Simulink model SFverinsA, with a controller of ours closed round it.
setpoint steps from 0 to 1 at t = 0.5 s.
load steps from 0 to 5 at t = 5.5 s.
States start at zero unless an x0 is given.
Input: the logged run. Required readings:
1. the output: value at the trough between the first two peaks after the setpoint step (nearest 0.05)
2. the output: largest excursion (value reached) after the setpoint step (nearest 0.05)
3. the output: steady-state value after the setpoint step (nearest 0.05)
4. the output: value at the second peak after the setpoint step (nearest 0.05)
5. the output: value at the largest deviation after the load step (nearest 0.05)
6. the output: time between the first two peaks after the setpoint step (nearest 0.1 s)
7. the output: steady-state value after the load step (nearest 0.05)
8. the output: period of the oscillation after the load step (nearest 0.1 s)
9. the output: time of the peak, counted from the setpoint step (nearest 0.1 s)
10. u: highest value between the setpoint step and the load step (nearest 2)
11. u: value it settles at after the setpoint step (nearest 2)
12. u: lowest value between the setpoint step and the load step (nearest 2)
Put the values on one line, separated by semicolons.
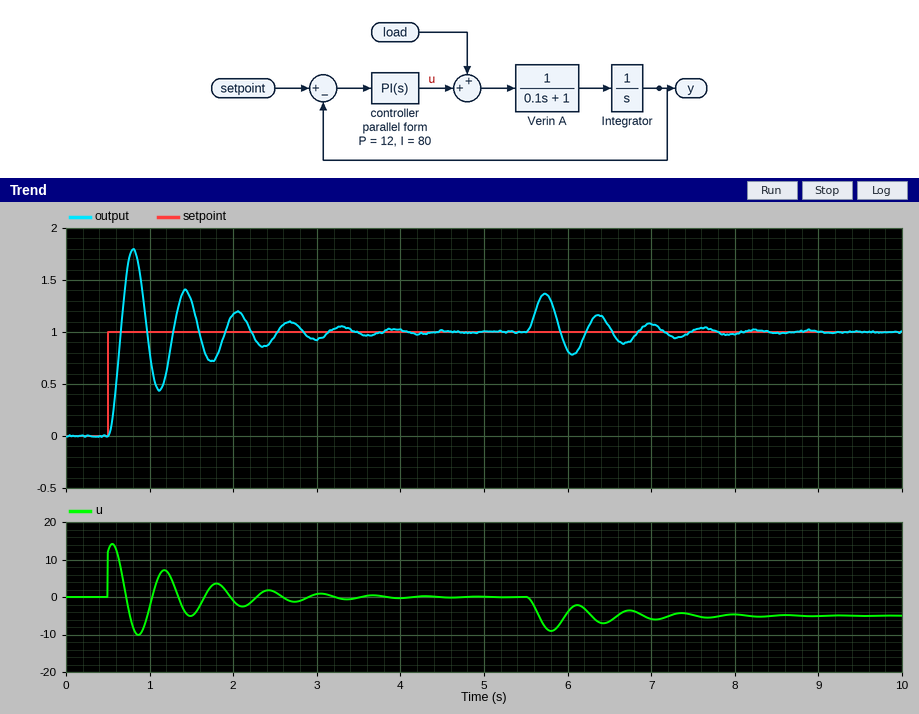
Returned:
0.45; 1.80; 1.00; 1.40; 1.35; 0.6 s; 1.00; 0.6 s; 0.3 s; 14; 0; -10
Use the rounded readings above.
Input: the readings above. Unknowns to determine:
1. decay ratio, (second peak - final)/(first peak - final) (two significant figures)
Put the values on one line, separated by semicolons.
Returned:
0.50
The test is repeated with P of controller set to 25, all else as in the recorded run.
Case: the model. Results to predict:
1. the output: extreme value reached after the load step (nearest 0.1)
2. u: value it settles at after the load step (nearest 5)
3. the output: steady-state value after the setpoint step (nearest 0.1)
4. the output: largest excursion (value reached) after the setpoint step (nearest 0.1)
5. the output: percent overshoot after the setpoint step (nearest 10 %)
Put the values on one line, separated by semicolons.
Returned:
1.2; -5; 1.0; 1.6; 60 %
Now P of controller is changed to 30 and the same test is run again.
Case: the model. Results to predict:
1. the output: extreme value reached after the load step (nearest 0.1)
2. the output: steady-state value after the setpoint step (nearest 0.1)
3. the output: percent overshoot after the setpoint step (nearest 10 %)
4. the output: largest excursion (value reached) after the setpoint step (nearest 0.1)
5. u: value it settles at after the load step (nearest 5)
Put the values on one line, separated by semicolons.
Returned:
1.2; 1.0; 60 %; 1.6; -5
